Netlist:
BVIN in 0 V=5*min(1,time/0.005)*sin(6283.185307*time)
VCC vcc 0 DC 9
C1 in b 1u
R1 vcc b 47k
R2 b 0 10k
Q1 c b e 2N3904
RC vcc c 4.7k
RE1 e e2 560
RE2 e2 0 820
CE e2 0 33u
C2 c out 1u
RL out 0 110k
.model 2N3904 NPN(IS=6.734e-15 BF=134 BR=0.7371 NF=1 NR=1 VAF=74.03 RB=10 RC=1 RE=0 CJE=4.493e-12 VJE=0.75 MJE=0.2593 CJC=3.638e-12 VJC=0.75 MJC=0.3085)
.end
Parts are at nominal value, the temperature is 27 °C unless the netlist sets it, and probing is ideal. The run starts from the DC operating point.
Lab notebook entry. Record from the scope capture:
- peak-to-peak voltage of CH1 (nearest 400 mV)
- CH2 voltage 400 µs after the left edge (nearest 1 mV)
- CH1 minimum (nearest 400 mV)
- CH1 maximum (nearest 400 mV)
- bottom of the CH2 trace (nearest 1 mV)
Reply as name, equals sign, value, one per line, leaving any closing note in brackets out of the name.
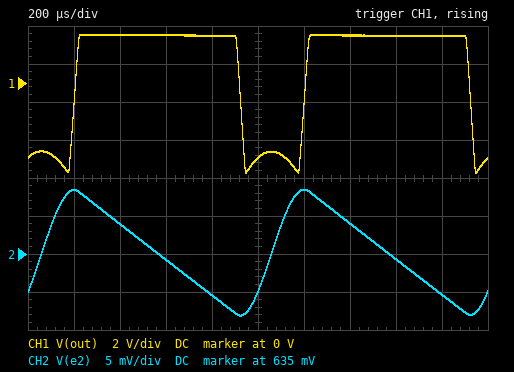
peak-to-peak voltage of CH1 = 7.2 V
CH2 voltage 400 µs after the left edge = 639 mV
CH1 minimum = -4.8 V
CH1 maximum = 2.4 V
bottom of the CH2 trace = 627 mV
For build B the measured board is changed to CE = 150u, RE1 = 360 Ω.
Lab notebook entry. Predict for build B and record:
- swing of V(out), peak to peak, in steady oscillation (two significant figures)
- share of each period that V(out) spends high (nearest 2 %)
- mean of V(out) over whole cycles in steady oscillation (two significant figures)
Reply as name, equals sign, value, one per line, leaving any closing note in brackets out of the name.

swing of V(out), peak to peak, in steady oscillation = 7.6 V
share of each period that V(out) spends high = 76 %
mean of V(out) over whole cycles in steady oscillation = 1.0 V
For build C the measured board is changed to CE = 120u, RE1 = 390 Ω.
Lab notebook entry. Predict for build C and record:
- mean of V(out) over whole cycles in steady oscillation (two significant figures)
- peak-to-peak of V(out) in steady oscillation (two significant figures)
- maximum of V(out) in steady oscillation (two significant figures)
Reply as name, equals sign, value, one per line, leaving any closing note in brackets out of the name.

mean of V(out) over whole cycles in steady oscillation = 950 mV
peak-to-peak of V(out) in steady oscillation = 7.5 V
maximum of V(out) in steady oscillation = 2.7 V
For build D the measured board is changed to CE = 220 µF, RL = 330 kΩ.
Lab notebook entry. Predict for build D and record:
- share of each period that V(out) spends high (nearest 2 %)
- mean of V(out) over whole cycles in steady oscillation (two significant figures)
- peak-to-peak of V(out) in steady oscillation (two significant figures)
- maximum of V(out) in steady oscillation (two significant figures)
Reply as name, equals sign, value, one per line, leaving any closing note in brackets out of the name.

share of each period that V(out) spends high = 72 %
mean of V(out) over whole cycles in steady oscillation = 940 mV
peak-to-peak of V(out) in steady oscillation = 7.4 V
maximum of V(out) in steady oscillation = 2.8 V
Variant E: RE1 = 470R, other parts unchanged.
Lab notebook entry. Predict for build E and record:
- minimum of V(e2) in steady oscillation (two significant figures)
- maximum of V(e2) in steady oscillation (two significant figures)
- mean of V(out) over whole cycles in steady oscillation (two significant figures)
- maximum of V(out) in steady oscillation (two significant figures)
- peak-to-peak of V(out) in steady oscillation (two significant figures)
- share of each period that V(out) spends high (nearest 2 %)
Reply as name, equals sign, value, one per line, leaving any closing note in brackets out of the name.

minimum of V(e2) in steady oscillation = 640 mV
maximum of V(e2) in steady oscillation = 660 mV
mean of V(out) over whole cycles in steady oscillation = 810 mV
maximum of V(out) in steady oscillation = 2.6 V
peak-to-peak of V(out) in steady oscillation = 7.4 V
share of each period that V(out) spends high = 74 %
